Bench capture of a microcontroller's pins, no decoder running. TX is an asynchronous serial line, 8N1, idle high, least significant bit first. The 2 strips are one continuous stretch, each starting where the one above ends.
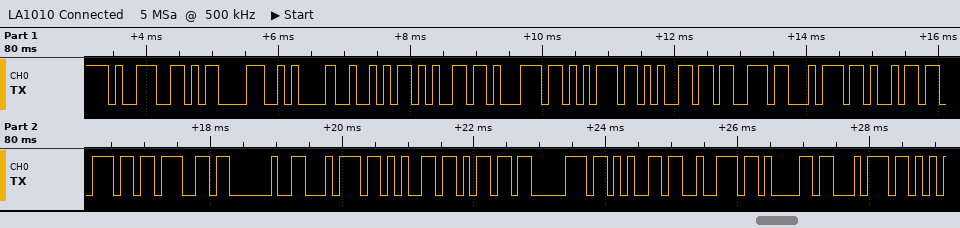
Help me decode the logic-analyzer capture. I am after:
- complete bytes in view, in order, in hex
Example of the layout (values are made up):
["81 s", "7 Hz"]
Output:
["39 0D 0A 52 65 71 75 65 73 74 69 6E 67 20 74 65 6D 70 65 72 61 74"]
